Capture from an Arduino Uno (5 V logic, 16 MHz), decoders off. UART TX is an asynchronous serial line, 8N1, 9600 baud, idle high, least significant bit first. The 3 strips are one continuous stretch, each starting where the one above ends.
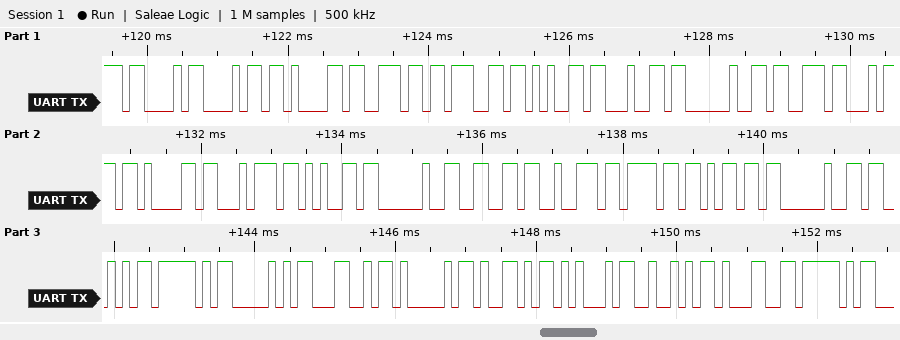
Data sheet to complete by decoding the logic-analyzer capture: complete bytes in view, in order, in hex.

43 68 61 6E 67 65 64 20 73 74 61 74 65 20 66 72 6F 6D 20 53 5F 50 4C 41 59 45 52 31 5F
